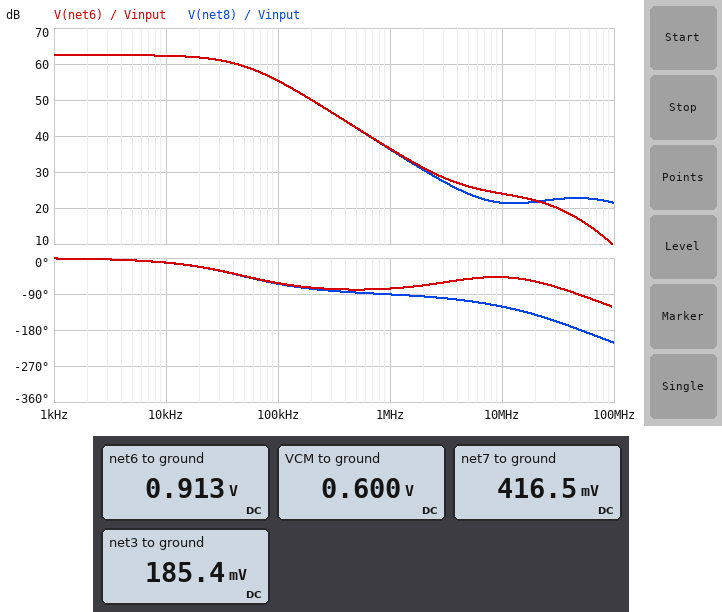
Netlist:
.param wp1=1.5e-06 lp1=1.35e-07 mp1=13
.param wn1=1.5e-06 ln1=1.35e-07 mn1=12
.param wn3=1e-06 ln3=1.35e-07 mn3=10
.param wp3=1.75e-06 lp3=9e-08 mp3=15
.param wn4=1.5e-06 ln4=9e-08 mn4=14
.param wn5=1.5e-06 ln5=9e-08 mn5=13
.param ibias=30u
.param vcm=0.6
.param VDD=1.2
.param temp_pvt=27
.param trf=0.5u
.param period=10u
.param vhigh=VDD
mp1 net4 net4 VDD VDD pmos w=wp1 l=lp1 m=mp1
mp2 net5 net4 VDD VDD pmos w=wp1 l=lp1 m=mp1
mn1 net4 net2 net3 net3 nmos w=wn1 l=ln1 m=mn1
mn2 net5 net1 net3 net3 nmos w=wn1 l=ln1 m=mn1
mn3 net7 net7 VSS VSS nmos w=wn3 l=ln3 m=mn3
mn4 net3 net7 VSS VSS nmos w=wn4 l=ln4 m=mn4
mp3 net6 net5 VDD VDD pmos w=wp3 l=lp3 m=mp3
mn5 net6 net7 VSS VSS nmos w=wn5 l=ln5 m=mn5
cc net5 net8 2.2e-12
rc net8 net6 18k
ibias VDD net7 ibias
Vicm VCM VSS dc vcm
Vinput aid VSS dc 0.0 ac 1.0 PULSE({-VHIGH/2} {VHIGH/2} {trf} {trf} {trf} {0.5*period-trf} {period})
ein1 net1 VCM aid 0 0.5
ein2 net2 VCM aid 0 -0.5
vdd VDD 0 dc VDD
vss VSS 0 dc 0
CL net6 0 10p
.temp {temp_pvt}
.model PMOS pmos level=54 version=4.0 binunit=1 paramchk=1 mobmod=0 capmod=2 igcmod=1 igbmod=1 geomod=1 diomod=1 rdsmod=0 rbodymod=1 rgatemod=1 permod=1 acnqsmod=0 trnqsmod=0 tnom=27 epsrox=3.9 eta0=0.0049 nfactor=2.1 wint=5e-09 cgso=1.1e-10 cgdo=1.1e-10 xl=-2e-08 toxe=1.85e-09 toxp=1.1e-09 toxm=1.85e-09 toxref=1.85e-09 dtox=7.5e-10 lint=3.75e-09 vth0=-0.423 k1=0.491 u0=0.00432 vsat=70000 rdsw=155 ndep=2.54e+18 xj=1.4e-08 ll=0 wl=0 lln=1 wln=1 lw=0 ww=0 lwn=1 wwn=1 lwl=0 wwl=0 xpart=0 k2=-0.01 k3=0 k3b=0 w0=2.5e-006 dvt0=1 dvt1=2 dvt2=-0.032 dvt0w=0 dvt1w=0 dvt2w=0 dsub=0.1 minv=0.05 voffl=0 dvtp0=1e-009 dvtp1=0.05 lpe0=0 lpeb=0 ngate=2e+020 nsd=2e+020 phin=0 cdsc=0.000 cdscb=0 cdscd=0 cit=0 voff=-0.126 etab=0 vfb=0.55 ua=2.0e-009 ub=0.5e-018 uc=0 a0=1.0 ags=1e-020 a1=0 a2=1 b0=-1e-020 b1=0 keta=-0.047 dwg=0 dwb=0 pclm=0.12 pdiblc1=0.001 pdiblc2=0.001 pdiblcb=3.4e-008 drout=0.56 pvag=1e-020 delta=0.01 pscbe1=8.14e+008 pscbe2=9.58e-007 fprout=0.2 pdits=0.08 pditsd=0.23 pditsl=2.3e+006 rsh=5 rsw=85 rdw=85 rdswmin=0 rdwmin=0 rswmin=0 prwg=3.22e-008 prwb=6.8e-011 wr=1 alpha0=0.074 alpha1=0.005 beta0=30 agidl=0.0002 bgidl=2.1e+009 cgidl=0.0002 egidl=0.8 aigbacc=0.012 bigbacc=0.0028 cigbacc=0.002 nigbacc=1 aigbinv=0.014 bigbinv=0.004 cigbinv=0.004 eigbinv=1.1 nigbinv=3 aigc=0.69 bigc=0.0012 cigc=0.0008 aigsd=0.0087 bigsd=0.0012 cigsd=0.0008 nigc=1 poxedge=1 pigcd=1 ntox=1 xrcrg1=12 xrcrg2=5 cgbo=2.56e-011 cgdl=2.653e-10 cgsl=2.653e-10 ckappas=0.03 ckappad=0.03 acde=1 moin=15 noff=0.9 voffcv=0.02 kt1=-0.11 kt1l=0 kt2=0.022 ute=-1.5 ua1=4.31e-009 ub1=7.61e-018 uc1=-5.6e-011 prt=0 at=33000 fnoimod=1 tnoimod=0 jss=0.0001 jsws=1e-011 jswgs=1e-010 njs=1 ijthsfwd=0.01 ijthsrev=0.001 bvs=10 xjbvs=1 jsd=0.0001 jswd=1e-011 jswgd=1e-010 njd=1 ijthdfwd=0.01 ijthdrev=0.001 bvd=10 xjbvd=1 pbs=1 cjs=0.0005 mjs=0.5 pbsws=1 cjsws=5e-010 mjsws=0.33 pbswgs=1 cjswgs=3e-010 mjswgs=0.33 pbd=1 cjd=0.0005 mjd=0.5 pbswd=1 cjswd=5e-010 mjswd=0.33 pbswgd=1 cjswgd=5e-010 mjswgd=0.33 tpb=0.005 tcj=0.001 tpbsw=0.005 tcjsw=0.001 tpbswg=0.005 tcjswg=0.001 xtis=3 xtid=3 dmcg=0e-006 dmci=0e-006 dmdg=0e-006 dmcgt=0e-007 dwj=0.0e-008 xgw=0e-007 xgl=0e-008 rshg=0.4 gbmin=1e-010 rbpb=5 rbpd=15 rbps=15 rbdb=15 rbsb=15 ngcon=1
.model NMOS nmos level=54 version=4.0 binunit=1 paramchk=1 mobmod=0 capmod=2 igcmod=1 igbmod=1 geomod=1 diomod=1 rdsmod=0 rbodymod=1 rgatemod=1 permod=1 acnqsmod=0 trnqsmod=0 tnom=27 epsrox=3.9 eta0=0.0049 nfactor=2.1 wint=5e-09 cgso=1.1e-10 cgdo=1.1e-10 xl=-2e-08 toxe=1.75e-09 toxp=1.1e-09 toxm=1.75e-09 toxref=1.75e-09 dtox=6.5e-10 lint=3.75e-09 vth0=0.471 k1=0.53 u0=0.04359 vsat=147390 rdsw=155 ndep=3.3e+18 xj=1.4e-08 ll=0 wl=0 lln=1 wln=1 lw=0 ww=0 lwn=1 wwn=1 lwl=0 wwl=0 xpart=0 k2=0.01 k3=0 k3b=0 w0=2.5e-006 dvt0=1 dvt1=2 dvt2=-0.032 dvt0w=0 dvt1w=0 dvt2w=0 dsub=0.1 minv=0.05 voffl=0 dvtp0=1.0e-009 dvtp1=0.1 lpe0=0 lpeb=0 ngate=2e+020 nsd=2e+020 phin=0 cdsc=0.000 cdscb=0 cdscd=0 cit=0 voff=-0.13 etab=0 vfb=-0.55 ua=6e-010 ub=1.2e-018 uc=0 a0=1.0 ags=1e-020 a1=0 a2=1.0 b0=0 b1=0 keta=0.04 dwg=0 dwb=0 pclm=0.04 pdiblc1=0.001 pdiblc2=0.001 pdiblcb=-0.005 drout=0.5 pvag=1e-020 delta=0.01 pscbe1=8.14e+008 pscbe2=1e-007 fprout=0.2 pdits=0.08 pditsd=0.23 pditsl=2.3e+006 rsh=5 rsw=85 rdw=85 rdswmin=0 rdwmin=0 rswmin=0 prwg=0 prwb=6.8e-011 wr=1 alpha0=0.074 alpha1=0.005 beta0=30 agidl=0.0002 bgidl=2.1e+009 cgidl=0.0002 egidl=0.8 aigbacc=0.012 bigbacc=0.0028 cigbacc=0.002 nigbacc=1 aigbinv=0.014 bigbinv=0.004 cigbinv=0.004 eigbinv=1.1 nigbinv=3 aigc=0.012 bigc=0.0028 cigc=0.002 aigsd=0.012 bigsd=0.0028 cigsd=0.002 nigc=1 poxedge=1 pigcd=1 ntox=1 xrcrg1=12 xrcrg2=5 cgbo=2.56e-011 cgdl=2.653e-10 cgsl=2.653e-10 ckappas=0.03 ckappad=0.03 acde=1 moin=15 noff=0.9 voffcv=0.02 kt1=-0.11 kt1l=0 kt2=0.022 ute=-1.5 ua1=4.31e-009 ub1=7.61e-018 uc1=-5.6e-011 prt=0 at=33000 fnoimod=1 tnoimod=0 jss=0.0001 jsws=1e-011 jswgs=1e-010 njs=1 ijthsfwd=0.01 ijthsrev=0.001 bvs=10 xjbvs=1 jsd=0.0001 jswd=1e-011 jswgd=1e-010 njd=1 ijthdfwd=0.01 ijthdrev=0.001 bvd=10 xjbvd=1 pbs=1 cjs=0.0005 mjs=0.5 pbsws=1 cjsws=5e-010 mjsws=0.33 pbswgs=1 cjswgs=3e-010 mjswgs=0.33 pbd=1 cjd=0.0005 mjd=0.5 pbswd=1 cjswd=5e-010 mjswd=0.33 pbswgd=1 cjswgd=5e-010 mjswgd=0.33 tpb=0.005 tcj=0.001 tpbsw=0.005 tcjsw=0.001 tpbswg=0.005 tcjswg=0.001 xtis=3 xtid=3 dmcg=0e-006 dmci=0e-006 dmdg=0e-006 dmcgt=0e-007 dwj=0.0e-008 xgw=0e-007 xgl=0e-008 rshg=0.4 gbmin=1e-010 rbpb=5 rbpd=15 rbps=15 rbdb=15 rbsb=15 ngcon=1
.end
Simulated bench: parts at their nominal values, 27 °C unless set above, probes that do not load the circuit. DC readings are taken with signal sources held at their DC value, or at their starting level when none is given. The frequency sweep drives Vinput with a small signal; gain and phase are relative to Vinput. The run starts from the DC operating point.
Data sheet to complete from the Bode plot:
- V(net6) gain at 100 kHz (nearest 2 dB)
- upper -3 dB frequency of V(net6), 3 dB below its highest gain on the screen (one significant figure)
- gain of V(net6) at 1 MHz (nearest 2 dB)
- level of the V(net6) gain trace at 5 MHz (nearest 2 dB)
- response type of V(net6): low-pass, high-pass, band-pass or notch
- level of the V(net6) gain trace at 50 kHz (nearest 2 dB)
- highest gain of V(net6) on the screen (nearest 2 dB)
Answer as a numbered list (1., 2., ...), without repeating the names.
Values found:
1. 56 dB
2. 50 kHz
3. 36 dB
4. 26 dB
5. low-pass
6. 60 dB
7. 62 dB
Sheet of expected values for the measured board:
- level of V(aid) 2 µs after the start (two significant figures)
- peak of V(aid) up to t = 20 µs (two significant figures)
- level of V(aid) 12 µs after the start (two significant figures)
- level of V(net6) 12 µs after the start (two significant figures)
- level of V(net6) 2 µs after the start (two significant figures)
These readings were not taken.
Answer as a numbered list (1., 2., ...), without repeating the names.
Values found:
1. 600 mV
2. 600 mV
3. 600 mV
4. 1.2 V
5. 1.2 V
